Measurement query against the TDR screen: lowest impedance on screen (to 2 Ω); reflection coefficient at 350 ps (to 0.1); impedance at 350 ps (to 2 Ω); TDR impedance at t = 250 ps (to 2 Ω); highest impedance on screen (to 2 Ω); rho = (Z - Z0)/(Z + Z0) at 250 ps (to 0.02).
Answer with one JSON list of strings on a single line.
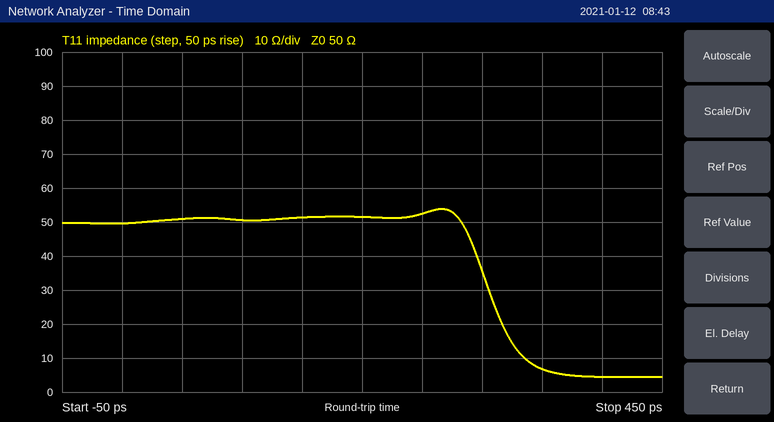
["4 Ω", "-0.8", "6 Ω", "52 Ω", "54 Ω", "+0.02"]
